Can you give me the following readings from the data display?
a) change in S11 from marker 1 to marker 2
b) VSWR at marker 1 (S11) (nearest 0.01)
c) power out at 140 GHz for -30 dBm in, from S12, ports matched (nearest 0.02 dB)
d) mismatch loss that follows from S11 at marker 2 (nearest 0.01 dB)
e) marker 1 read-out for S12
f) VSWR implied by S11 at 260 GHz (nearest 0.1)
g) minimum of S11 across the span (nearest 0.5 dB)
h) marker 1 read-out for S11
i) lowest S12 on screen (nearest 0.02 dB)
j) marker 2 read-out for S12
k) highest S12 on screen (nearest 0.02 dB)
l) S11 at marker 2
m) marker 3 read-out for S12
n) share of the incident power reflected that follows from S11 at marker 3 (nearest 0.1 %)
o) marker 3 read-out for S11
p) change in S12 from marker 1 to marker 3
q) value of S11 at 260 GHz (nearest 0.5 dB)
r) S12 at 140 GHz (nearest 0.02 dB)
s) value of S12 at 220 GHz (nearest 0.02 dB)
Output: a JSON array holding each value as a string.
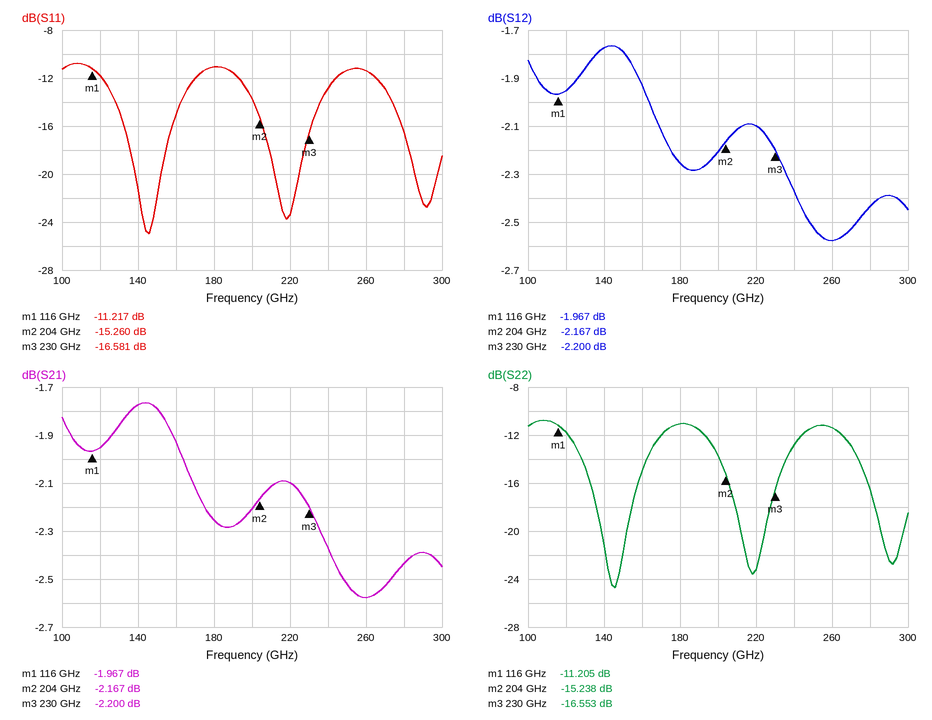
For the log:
["-4.043 dB", "1.76", "-31.78 dBm", "0.13 dB", "-1.967 dB", "1.7", "-25.0 dB", "-11.217 dB", "-2.58 dB", "-2.167 dB", "-1.76 dB", "-15.260 dB", "-2.200 dB", "2.2 %", "-16.581 dB", "-0.233 dB", "-11.5 dB", "-1.78 dB", "-2.10 dB"]
